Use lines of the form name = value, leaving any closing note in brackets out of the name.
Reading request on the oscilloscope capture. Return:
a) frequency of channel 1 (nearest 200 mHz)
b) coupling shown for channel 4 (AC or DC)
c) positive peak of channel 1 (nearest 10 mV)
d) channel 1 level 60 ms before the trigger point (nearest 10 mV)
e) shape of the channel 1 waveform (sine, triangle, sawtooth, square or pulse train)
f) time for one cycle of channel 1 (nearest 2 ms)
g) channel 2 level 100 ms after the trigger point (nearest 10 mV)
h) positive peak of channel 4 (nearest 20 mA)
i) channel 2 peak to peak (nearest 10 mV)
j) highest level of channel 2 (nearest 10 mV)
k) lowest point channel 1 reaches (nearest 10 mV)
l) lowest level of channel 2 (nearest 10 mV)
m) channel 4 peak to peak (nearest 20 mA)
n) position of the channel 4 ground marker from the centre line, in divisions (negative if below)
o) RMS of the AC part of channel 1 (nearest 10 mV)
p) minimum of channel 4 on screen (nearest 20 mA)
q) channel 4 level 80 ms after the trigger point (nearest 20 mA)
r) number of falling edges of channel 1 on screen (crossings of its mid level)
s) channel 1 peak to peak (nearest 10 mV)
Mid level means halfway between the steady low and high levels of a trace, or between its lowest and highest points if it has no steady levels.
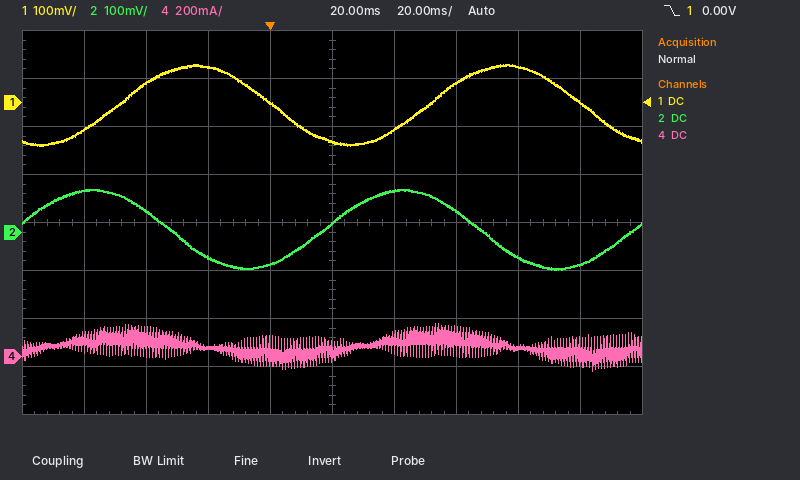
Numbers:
frequency of channel 1 = 10.0 Hz
coupling shown for channel 4 = DC
positive peak of channel 1 = 80 mV
channel 1 level 60 ms before the trigger point = -60 mV
shape of the channel 1 waveform = sine
time for one cycle of channel 1 = 100 ms
channel 2 level 100 ms after the trigger point = -70 mV
positive peak of channel 4 = 140 mA
channel 2 peak to peak = 170 mV
highest level of channel 2 = 90 mV
lowest point channel 1 reaches = -90 mV
lowest level of channel 2 = -80 mV
channel 4 peak to peak = 200 mA
position of the channel 4 ground marker from the centre line, in divisions = -2.8 div
RMS of the AC part of channel 1 = 60 mV
minimum of channel 4 on screen = -60 mA
channel 4 level 80 ms after the trigger point = 40 mA
number of falling edges of channel 1 on screen = 2
channel 1 peak to peak = 170 mV
